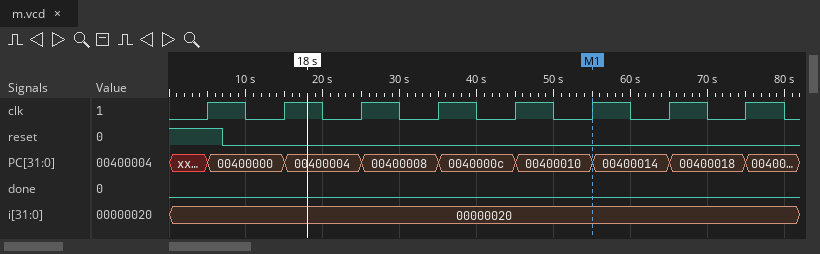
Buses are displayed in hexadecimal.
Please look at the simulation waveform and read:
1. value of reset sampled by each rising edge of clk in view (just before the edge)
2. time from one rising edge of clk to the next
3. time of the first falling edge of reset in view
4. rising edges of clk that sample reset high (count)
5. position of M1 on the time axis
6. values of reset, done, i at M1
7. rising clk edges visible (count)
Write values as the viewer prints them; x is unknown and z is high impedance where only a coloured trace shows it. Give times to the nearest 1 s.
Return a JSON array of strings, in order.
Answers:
["1 0 0 0 0 0 0 0", "10 s", "7 s", "1", "55 s", "reset=0, done=0, i=00000020", "8"]
